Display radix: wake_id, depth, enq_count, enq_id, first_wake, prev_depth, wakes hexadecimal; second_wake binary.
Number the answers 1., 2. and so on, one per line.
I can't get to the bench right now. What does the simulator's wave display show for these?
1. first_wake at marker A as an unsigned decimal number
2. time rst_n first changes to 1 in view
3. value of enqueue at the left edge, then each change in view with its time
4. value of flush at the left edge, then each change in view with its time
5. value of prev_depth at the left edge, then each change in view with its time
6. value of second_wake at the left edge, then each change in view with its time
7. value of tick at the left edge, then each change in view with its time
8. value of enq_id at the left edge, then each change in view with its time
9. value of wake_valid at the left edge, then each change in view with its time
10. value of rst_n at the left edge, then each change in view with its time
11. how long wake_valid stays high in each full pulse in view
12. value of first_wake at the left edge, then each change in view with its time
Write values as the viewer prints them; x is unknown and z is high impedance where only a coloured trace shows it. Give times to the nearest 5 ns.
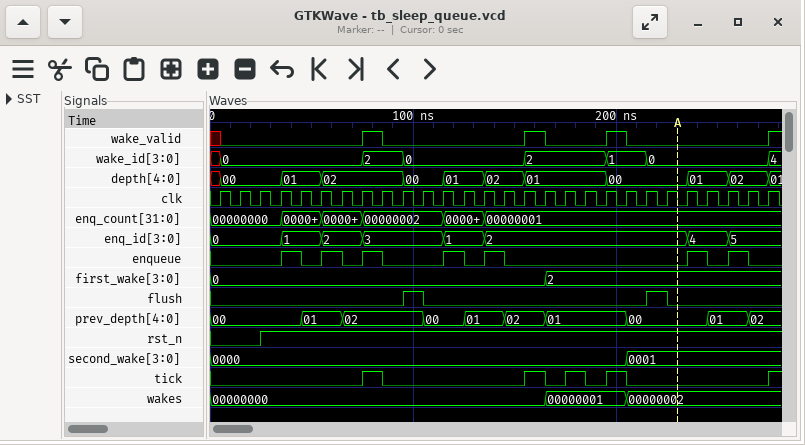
1. 2
2. 25 ns
3. 0, 1 at 35 ns, 0 at 45 ns, 1 at 55 ns, 0 at 65 ns, 1 at 75 ns, 0 at 85 ns, 1 at 115 ns, 0 at 125 ns, 1 at 135 ns, 0 at 145 ns, 1 at 235 ns, 0 at 245 ns, 1 at 255 ns, 0 at 265 ns
4. 0, 1 at 95 ns, 0 at 105 ns, 1 at 215 ns, 0 at 225 ns
5. 00, 01 at 45 ns, 02 at 65 ns, 00 at 105 ns, 01 at 125 ns, 02 at 145 ns, 01 at 165 ns, 00 at 205 ns, 01 at 245 ns, 02 at 265 ns
6. 0000, 0001 at 205 ns
7. 0, 1 at 75 ns, 0 at 85 ns, 1 at 155 ns, 0 at 165 ns, 1 at 175 ns, 0 at 185 ns, 1 at 195 ns, 0 at 205 ns, 1 at 275 ns
8. 0, 1 at 35 ns, 2 at 55 ns, 3 at 75 ns, 1 at 115 ns, 2 at 135 ns, 4 at 235 ns, 5 at 255 ns
9. x, 0 at 5 ns, 1 at 75 ns, 0 at 85 ns, 1 at 155 ns, 0 at 165 ns, 1 at 195 ns, 0 at 205 ns, 1 at 275 ns
10. 0, 1 at 25 ns
11. 10 ns, 10 ns, 10 ns
12. 0, 2 at 165 ns
